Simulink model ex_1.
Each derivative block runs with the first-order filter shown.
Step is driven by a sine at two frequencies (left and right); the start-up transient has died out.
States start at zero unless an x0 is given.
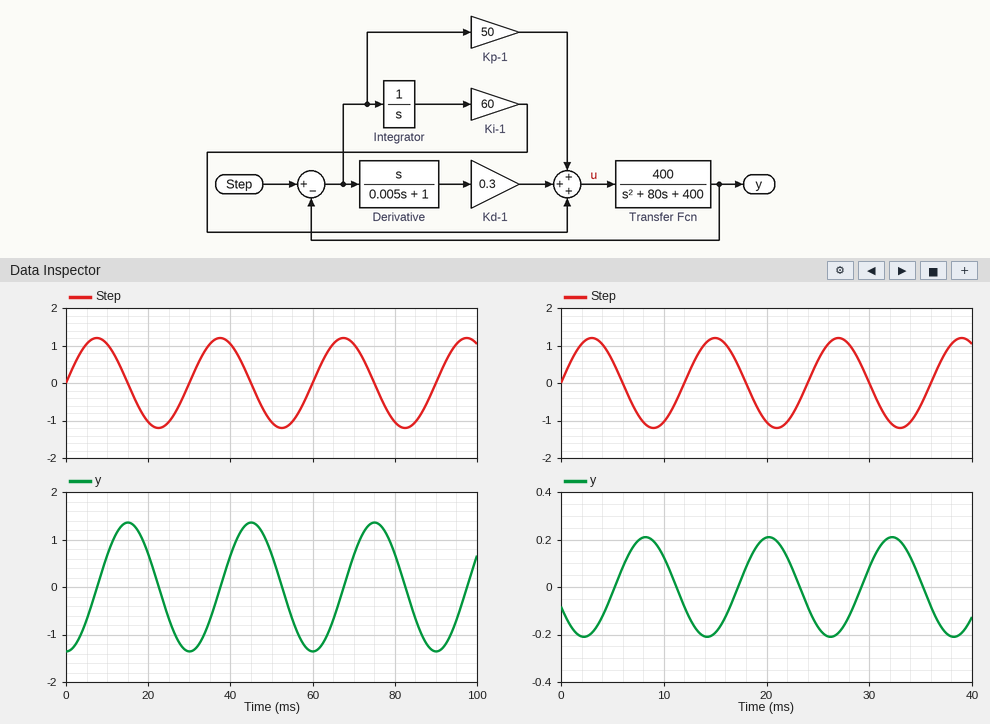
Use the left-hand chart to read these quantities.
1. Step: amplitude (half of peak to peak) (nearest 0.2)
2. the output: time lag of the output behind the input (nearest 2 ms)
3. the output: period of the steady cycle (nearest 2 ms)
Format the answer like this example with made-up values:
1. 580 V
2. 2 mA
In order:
1. 1.2
2. 8 ms
3. 30 ms
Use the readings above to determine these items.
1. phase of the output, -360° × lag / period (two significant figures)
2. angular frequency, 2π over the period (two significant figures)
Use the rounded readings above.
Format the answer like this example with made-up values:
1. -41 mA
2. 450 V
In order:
1. -96°
2. 0.21 rad/ms
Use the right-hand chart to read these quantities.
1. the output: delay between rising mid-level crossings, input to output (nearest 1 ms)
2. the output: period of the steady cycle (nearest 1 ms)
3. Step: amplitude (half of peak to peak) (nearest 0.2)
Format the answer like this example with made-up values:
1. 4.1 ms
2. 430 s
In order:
1. 5 ms
2. 12 ms
3. 1.2
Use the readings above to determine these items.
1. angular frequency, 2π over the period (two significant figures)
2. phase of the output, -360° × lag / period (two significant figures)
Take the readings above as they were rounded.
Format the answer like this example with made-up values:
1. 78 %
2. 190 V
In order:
1. 0.52 rad/ms
2. -150°
